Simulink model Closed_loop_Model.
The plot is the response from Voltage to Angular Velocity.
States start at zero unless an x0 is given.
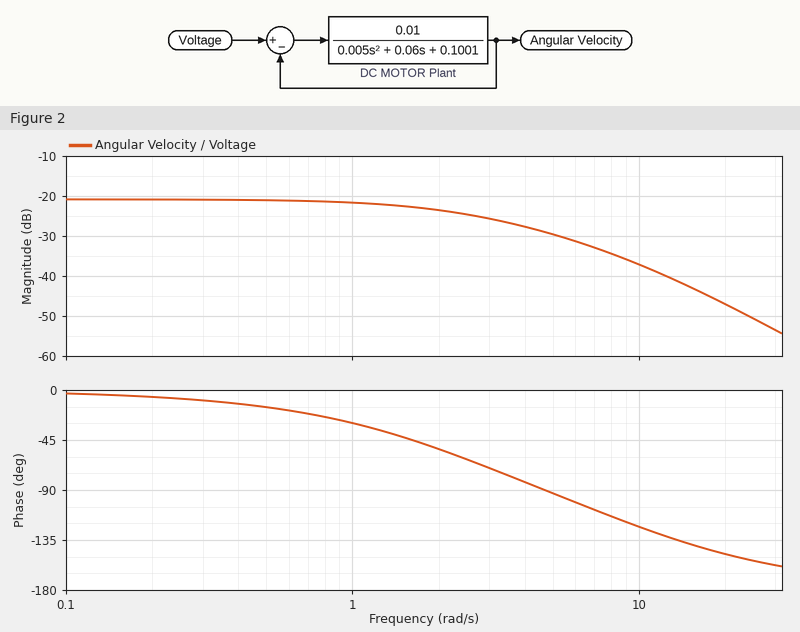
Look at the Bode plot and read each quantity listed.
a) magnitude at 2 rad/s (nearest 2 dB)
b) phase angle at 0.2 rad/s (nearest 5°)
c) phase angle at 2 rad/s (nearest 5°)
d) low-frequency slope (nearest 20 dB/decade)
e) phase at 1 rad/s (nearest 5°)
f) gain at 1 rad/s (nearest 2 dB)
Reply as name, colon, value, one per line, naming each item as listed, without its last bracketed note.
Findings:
magnitude at 2 rad/s: -24 dB
phase angle at 0.2 rad/s: -5°
phase angle at 2 rad/s: -55°
low-frequency slope: 0 dB/decade
phase at 1 rad/s: -30°
gain at 1 rad/s: -22 dB
